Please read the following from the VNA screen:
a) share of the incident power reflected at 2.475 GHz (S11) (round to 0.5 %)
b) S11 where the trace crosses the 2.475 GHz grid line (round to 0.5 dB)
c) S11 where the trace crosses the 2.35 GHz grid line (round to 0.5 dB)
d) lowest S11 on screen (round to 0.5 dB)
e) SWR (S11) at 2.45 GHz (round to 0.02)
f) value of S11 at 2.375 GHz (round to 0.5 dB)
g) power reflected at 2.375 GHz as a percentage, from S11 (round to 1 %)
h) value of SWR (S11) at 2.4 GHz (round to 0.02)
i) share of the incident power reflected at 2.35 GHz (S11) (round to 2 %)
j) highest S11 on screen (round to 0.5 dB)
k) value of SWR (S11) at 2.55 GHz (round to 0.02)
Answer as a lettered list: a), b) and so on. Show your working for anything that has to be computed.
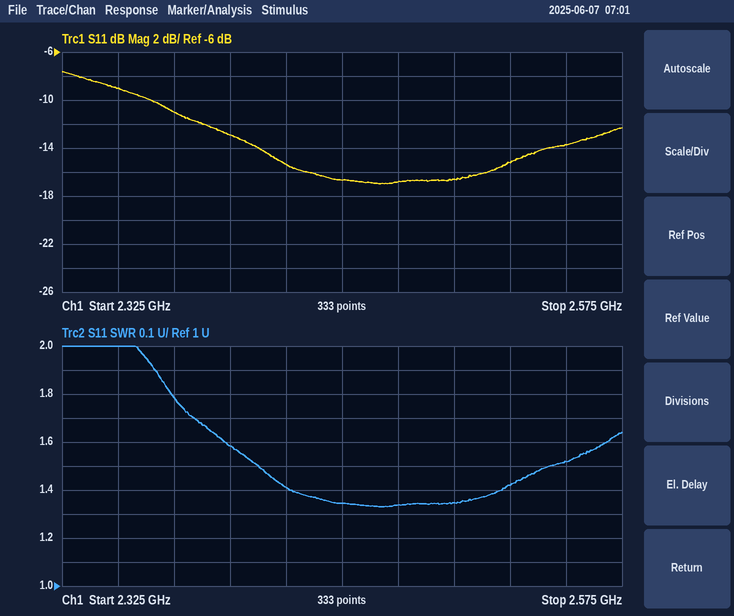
a) 10^(-17/10) ≈ 2.0 %
b) -17.0 dB
c) -9.0 dB
d) -17.0 dB
e) 1.34
f) -11.0 dB
g) 10^(-11/10) ≈ 8 %
h) 1.58
i) 10^(-9/10) ≈ 12.6 %, so 12 % to the nearest 2 %
j) -7.5 dB
k) 1.52
